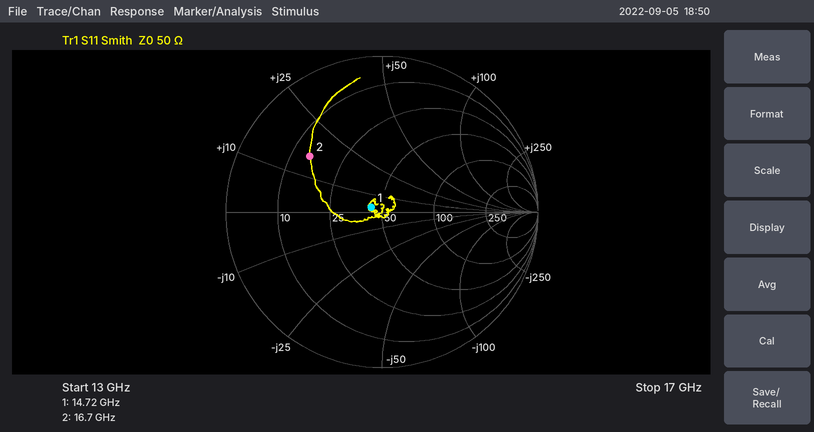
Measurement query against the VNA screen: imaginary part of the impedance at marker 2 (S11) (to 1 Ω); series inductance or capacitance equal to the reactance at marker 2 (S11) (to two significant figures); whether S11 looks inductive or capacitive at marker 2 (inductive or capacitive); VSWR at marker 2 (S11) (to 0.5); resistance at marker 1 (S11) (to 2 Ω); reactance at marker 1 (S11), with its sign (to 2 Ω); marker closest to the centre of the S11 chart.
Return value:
+16 Ω
150 pH
inductive
4.0
44 Ω
+2 Ω
marker 1
